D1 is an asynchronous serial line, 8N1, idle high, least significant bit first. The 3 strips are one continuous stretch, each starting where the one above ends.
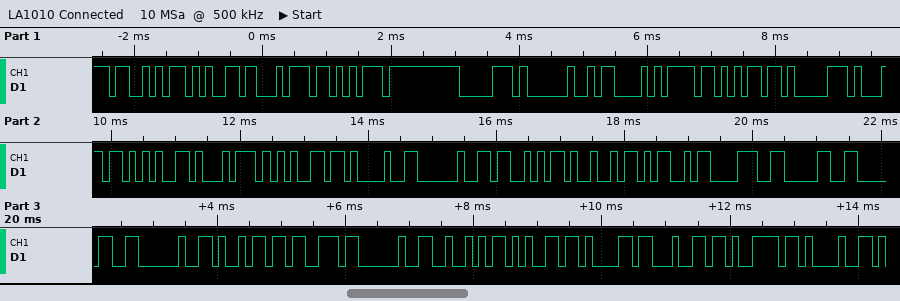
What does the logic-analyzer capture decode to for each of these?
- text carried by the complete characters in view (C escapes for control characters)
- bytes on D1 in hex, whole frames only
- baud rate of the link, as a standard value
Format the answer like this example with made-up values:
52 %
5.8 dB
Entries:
"Setup Complete! SIM800 is Ready!"
53 65 74 75 70 20 43 6F 6D 70 6C 65 74 65 21 20 53 49 4D 38 30 30 20 69 73 20 52 65 61 64 79 21
9600 baud
